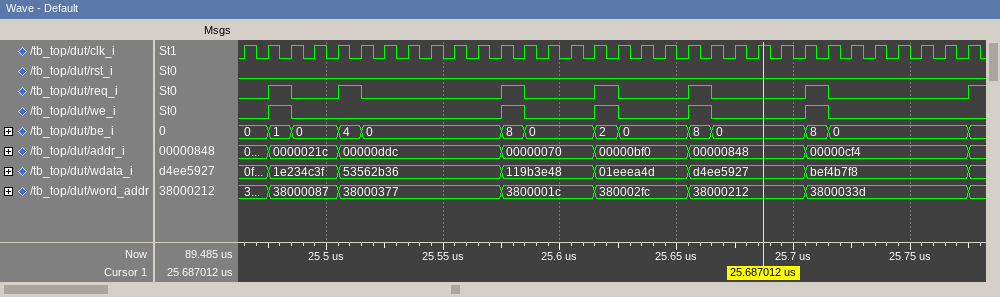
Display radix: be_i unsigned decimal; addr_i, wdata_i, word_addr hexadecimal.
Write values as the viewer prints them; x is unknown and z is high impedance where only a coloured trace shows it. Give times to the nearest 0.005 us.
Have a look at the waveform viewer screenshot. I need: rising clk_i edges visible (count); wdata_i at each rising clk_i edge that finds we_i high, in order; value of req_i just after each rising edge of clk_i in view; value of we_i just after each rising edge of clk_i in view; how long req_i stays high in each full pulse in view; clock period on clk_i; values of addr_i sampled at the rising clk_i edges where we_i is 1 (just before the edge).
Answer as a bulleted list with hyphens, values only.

- 32
- 1e234c3f, 119b3e48, 01eeea4d, d4ee5927, bef4b7f8
- 0 1 0 0 1 0 0 0 0 0 0 1 0 0 0 1 0 0 0 1 0 0 0 0 1 0 0 0 0 0 0 1
- 0 1 0 0 0 0 0 0 0 0 0 1 0 0 0 1 0 0 0 1 0 0 0 0 1 0 0 0 0 0 0 0
- 0.01 us, 0.01 us, 0.01 us, 0.01 us, 0.01 us, 0.01 us
- 0.01 us
- 0000021c, 00000070, 00000bf0, 00000848, 00000cf4
